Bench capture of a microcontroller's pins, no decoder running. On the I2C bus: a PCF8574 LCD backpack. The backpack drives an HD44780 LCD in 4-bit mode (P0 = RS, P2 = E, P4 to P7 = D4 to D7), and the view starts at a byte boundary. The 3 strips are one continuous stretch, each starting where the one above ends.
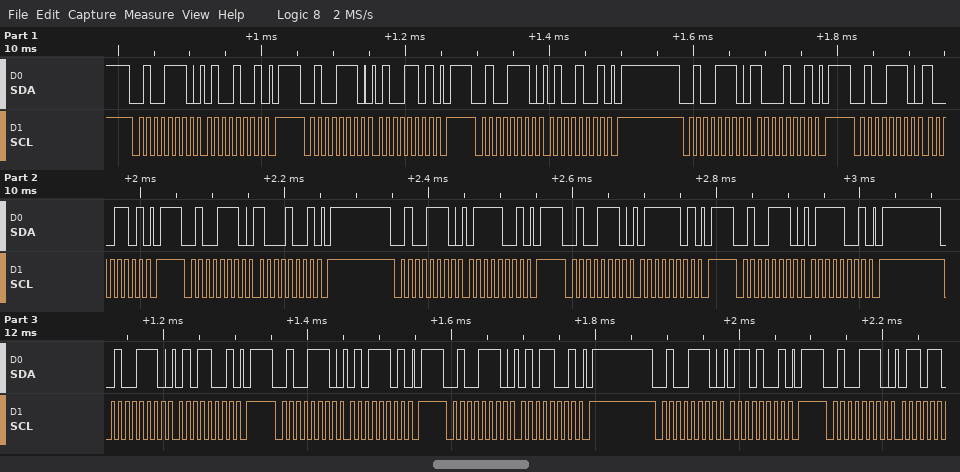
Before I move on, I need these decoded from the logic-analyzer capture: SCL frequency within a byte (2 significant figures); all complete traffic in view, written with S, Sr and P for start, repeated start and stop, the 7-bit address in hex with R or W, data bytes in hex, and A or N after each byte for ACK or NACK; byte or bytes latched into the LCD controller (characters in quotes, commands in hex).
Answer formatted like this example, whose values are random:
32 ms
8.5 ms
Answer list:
100 kHz
S 27W A 49 A P S 27W A 4D A P S 27W A 49 A P S 27W A 89 A P S 27W A 8D A P S 27W A 89 A P S 27W A 79 A P S 27W A 7D A P S 27W A 79 A P S 27W A 59 A P S 27W A 5D A P S 27W A 59 A P S 27W A 69 A P S 27W A
'H' 'u'
